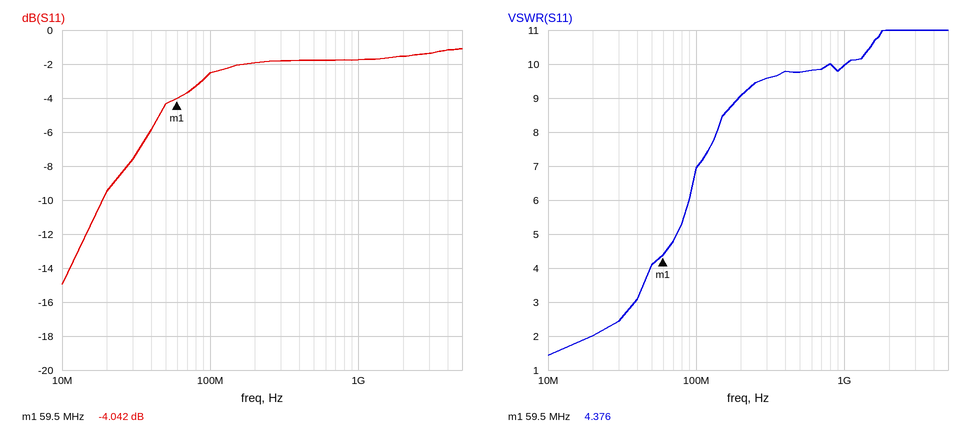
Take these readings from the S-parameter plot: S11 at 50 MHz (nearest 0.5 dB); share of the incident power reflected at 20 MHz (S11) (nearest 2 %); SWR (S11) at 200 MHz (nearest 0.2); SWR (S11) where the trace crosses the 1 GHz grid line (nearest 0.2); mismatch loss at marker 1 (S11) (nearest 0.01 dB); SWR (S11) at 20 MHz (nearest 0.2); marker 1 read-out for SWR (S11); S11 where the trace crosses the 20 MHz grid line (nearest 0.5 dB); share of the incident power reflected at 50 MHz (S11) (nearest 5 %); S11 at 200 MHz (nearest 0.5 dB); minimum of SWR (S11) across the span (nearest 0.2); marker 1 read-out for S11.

-4.5 dB
12 %
9.0
10.0
2.18 dB
2.0
4.376
-9.5 dB
35 %
-2.0 dB
1.4
-4.042 dB
